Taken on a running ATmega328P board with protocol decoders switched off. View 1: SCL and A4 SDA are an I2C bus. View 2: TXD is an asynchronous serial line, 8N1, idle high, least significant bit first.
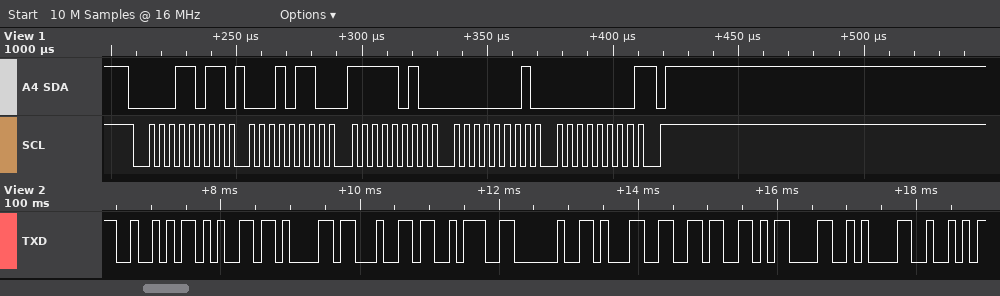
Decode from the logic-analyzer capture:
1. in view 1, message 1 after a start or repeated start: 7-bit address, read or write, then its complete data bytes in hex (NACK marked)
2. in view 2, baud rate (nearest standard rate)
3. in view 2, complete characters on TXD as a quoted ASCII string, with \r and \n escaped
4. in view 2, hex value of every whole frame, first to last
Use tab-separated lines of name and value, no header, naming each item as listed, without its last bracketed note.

in view 1, message 1 after a start or repeated start: 7-bit address, read or write, then its complete data bytes in hex	0x0D read: 16 FA 01 00 NACK
in view 2, baud rate	9600 baud
in view 2, complete characters on TXD as a quoted ASCII string, with \r and \n escaped	"Read: 16\r\nR"
in view 2, hex value of every whole frame, first to last	0x52 0x65 0x61 0x64 0x3A 0x20 0x31 0x36 0x0D 0x0A 0x52
